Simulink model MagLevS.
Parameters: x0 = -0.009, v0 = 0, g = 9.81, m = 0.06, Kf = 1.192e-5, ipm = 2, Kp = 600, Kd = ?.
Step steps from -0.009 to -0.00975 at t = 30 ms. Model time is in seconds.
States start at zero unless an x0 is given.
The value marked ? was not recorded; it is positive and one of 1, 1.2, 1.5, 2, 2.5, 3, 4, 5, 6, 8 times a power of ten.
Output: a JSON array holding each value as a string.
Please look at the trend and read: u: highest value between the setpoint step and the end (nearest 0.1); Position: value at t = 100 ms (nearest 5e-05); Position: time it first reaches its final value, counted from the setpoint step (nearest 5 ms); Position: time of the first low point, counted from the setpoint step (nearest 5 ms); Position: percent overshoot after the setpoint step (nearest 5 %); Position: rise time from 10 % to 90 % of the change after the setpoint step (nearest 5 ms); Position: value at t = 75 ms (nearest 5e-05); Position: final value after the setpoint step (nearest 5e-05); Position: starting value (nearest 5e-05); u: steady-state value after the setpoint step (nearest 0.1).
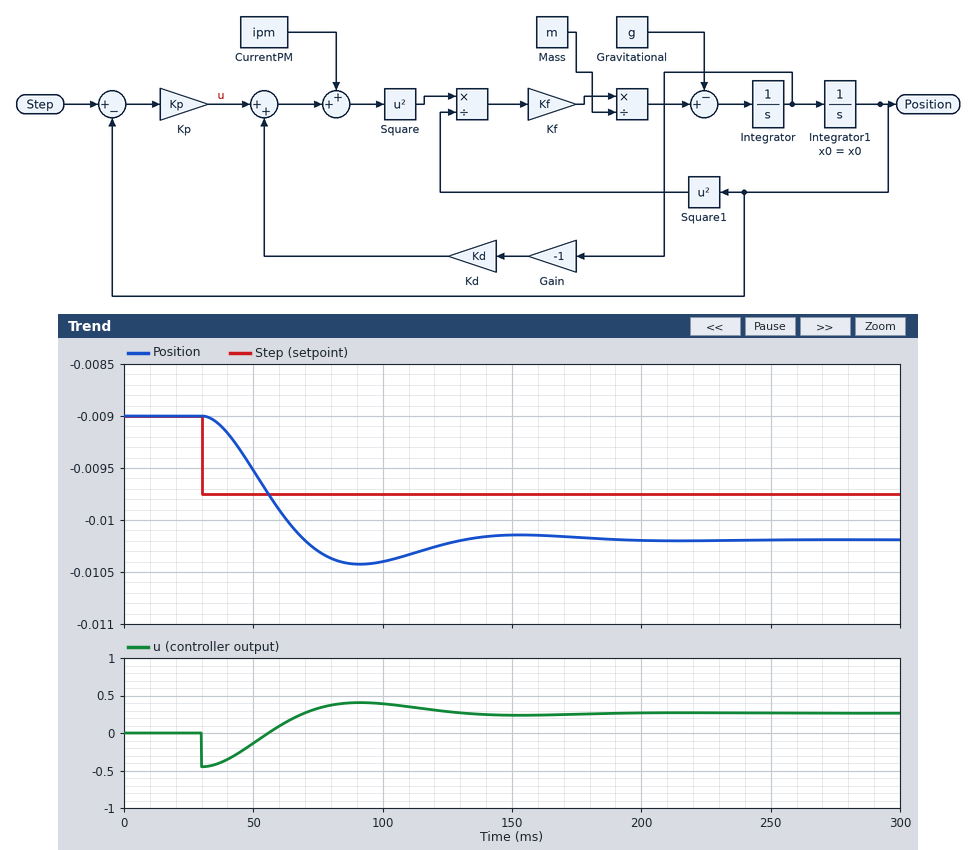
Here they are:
["0.4", "-0.01040", "40 ms", "60 ms", "20 %", "25 ms", "-0.01030", "-0.01020", "-0.00900", "0.3"]
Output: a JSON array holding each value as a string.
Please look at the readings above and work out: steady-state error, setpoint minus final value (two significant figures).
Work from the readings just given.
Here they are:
["0.00045"]
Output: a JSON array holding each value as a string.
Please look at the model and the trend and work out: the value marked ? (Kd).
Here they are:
["6"]
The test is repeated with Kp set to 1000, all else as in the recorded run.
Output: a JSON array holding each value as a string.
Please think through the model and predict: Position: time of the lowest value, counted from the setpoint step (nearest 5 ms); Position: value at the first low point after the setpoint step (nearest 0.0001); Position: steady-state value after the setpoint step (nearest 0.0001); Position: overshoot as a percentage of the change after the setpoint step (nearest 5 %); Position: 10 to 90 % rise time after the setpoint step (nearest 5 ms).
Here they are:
["40 ms", "-0.0103", "-0.0100", "35 %", "15 ms"]
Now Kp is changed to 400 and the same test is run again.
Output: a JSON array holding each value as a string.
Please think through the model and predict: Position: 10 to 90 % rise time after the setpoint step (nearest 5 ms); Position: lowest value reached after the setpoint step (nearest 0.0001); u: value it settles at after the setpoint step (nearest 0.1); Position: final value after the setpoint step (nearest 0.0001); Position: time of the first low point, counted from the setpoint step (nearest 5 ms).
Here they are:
["50 ms", "-0.0108", "0.4", "-0.0107", "105 ms"]
